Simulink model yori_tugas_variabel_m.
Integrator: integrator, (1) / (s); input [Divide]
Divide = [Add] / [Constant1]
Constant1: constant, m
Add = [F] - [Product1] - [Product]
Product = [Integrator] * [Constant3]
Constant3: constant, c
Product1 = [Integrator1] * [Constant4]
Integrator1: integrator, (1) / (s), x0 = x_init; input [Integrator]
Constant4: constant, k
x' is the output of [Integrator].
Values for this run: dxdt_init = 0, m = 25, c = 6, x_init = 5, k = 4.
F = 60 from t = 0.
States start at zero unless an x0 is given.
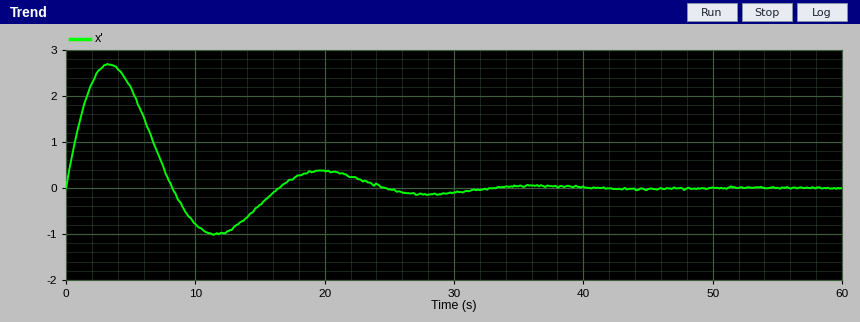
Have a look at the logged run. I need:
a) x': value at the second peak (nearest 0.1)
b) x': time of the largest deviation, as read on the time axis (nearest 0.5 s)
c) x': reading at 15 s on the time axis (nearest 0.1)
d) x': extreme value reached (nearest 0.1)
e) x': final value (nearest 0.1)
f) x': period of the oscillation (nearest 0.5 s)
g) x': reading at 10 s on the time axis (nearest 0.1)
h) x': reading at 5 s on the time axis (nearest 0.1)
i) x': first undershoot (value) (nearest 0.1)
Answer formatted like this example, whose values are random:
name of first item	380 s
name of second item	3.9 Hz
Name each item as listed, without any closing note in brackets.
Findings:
x': value at the second peak	0.4
x': time of the largest deviation, as read on the time axis	3.5 s
x': reading at 15 s on the time axis	-0.4
x': extreme value reached	2.7
x': final value	0.0
x': period of the oscillation	16.5 s
x': reading at 10 s on the time axis	-0.8
x': reading at 5 s on the time axis	2.2
x': first undershoot (value)	-1.0
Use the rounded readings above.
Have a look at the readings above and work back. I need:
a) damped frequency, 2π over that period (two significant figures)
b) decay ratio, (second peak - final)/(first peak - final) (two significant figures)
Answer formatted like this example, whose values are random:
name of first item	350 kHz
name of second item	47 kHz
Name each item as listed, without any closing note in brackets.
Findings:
damped frequency, 2π over that period	0.38 rad/s
decay ratio, (second peak - final)/(first peak - final)	0.15
